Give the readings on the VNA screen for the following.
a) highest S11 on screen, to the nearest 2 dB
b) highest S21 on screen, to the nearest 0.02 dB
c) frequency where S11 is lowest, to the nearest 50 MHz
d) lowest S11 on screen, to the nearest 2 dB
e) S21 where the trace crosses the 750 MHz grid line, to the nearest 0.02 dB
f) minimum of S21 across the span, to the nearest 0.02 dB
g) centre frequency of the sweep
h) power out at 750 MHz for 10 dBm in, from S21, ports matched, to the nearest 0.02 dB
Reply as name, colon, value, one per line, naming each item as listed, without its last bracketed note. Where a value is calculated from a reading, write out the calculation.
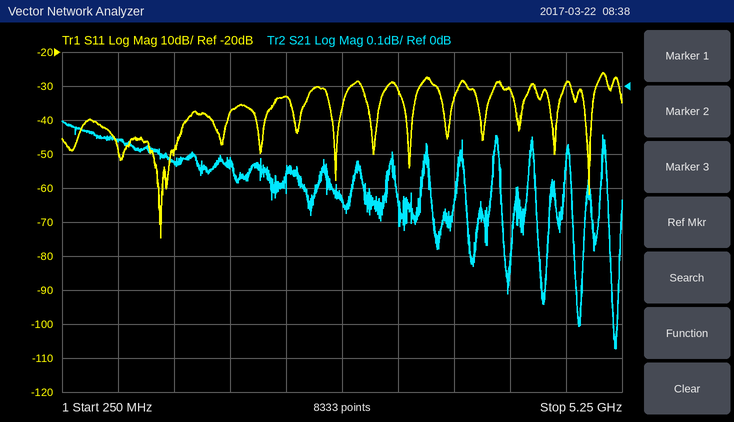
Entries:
highest S11 on screen, to the nearest 2 dB: -26 dB
highest S21 on screen, to the nearest 0.02 dB: -0.10 dB
frequency where S11 is lowest, to the nearest 50 MHz: 1.15 GHz
lowest S11 on screen, to the nearest 2 dB: -74 dB
S21 where the trace crosses the 750 MHz grid line, to the nearest 0.02 dB: -0.16 dB
minimum of S21 across the span, to the nearest 0.02 dB: -0.78 dB
centre frequency of the sweep: 2.75 GHz
power out at 750 MHz for 10 dBm in, from S21, ports matched, to the nearest 0.02 dB: 10 dBm + (-0.16 dB) = 9.84 dBm
